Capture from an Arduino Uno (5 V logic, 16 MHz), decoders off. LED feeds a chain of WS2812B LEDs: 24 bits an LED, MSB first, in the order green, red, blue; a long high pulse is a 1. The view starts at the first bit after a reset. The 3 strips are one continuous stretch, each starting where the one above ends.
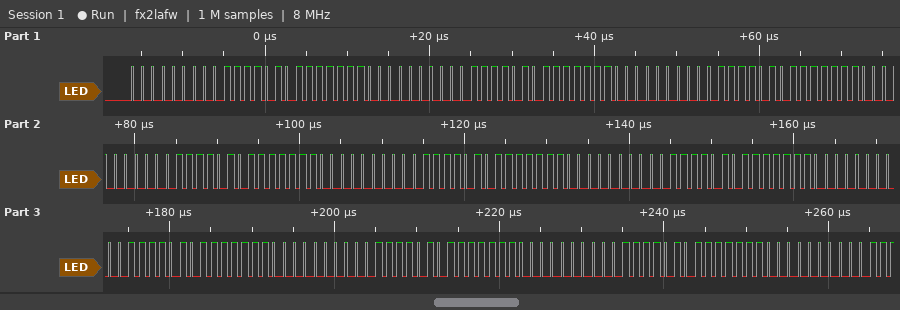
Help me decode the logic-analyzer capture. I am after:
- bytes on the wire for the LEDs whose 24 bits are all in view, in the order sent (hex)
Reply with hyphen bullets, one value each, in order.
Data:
- 00 7A FE 00 7A FE 00 7A FE 00 7A FE 00 7A FE 00 7A FE 00 7A FE 00 7A FE 00 7A FE
